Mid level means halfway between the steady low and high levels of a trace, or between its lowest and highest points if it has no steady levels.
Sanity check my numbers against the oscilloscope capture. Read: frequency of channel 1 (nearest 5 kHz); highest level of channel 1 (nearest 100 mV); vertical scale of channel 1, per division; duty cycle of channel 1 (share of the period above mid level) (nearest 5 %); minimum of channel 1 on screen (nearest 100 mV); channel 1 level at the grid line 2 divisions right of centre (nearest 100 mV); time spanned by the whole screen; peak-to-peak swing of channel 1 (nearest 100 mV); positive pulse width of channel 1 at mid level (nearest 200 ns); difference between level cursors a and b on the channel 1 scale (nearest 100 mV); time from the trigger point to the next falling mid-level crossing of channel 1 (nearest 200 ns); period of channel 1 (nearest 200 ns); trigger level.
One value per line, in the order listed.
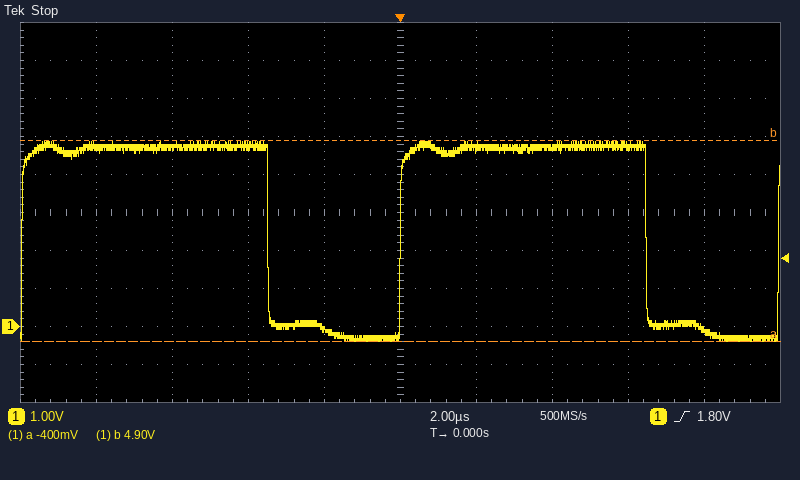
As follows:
100 kHz
4.9 V
1 V
65 %
-400 mV
4.7 V
20 µs
5.3 V
6.4 µs
5.3 V
6.4 µs
10.0 µs
1.80 V
